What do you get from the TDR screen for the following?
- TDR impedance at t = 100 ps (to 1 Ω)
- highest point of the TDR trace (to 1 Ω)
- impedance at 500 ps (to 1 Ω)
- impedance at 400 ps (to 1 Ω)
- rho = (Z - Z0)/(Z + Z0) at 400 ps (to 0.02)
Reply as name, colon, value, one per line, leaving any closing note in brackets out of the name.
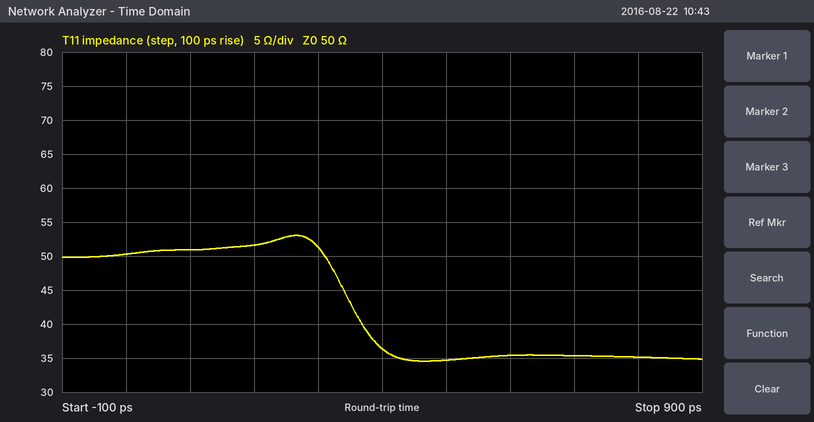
TDR impedance at t = 100 ps: 51 Ω
highest point of the TDR trace: 53 Ω
impedance at 500 ps: 35 Ω
impedance at 400 ps: 36 Ω
rho = (Z - Z0)/(Z + Z0) at 400 ps: -0.16
